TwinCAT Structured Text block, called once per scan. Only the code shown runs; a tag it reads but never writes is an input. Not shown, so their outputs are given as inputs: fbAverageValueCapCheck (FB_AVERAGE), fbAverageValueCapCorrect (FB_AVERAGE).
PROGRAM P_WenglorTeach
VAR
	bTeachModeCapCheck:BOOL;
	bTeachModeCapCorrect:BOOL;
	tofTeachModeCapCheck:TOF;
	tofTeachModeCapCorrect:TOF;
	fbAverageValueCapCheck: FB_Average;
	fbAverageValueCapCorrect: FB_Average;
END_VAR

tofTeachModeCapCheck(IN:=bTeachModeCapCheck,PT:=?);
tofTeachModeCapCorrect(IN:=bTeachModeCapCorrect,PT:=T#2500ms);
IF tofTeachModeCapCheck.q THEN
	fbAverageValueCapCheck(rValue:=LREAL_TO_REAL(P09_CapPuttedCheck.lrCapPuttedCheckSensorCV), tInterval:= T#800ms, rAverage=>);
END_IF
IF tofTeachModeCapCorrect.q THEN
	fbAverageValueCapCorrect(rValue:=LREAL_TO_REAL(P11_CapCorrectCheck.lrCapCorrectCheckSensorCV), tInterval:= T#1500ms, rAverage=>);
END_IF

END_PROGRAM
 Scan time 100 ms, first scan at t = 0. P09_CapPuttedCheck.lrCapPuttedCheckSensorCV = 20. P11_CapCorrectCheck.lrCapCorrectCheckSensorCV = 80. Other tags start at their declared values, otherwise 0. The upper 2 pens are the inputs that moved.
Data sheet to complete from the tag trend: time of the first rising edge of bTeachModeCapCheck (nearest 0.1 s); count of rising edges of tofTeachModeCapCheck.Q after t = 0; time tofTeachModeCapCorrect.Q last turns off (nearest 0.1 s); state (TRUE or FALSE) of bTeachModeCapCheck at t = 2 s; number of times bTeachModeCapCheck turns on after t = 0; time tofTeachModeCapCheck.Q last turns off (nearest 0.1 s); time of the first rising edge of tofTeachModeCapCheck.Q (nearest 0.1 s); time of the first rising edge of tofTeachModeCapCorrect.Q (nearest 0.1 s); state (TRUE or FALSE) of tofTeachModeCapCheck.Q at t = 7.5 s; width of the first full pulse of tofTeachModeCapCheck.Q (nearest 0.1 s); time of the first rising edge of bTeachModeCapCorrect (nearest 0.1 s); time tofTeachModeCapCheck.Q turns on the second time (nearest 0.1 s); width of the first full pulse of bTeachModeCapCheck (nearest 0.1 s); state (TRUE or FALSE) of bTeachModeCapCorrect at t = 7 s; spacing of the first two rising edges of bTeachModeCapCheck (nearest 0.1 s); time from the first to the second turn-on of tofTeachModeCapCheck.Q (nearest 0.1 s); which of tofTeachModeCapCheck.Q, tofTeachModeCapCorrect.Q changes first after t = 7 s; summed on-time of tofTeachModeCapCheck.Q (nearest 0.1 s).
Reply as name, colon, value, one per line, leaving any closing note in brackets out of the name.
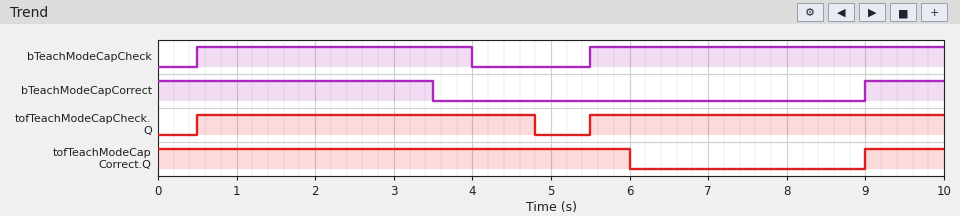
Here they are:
time of the first rising edge of bTeachModeCapCheck: 0.5 s
count of rising edges of tofTeachModeCapCheck.Q after t = 0: 2
time tofTeachModeCapCorrect.Q last turns off: 6.0 s
state (TRUE or FALSE) of bTeachModeCapCheck at t = 2 s: TRUE
number of times bTeachModeCapCheck turns on after t = 0: 2
time tofTeachModeCapCheck.Q last turns off: 4.8 s
time of the first rising edge of tofTeachModeCapCheck.Q: 0.5 s
time of the first rising edge of tofTeachModeCapCorrect.Q: 9.0 s
state (TRUE or FALSE) of tofTeachModeCapCheck.Q at t = 7.5 s: TRUE
width of the first full pulse of tofTeachModeCapCheck.Q: 4.3 s
time of the first rising edge of bTeachModeCapCorrect: 9.0 s
time tofTeachModeCapCheck.Q turns on the second time: 5.5 s
width of the first full pulse of bTeachModeCapCheck: 3.5 s
state (TRUE or FALSE) of bTeachModeCapCorrect at t = 7 s: FALSE
spacing of the first two rising edges of bTeachModeCapCheck: 5.0 s
time from the first to the second turn-on of tofTeachModeCapCheck.Q: 5.0 s
which of tofTeachModeCapCheck.Q, tofTeachModeCapCorrect.Q changes first after t = 7 s: tofTeachModeCapCorrect.Q
summed on-time of tofTeachModeCapCheck.Q: 8.8 s
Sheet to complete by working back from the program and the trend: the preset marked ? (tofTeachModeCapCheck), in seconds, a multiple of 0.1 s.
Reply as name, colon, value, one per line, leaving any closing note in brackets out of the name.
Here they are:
the preset marked ? (tofTeachModeCapCheck), in seconds, a multiple of 0.1 s: 0.8 s
